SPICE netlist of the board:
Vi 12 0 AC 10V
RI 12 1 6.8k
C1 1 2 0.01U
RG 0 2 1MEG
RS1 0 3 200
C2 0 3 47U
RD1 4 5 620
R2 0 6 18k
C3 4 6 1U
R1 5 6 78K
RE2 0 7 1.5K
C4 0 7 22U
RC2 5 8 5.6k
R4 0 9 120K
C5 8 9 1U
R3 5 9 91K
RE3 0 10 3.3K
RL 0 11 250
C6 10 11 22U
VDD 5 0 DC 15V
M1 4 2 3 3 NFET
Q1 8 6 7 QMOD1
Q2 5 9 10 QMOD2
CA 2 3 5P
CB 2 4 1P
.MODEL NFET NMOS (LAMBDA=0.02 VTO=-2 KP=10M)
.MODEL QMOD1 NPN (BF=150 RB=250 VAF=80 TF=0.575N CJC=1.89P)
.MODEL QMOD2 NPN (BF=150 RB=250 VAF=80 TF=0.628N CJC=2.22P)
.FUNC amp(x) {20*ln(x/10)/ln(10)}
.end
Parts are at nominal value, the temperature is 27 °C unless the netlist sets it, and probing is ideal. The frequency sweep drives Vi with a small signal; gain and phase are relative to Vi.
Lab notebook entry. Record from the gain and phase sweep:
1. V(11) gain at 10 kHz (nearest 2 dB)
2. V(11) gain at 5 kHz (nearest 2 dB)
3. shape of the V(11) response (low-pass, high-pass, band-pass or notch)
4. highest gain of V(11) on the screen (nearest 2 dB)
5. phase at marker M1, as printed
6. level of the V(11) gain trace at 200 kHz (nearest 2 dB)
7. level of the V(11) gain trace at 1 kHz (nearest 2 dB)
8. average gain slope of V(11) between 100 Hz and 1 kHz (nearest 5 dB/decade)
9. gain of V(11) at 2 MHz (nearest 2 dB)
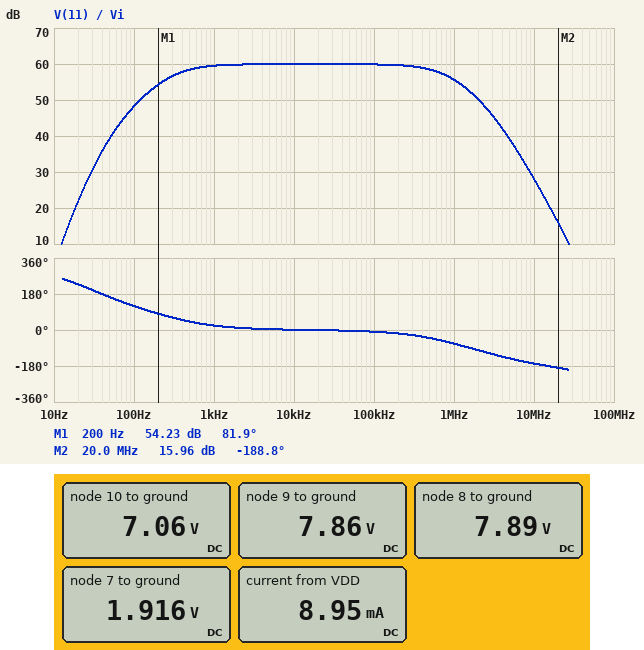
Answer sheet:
60 dB
60 dB
band-pass
60 dB
81.9 deg
60 dB
60 dB
10 dB/decade
50 dB
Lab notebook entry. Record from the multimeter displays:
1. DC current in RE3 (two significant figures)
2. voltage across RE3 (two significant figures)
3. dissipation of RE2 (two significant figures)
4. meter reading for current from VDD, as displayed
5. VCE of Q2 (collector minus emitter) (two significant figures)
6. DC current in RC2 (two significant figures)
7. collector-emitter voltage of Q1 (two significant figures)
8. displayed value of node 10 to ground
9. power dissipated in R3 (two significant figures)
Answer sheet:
2.1 mA
7.1 V
2.4 mW
8.95 mA
7.9 V
1.3 mA
6.0 V
7.06 V
560 µW
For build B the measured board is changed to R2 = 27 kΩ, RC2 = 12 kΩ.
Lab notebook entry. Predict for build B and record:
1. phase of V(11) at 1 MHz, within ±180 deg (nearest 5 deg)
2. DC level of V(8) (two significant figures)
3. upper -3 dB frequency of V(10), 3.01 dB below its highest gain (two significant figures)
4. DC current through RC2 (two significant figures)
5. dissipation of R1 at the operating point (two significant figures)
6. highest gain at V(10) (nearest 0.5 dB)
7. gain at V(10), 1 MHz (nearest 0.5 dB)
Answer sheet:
-20 deg
1.8 V
2.9 MHz
1.1 mA
2.0 mW
9.0 dB
8.5 dB
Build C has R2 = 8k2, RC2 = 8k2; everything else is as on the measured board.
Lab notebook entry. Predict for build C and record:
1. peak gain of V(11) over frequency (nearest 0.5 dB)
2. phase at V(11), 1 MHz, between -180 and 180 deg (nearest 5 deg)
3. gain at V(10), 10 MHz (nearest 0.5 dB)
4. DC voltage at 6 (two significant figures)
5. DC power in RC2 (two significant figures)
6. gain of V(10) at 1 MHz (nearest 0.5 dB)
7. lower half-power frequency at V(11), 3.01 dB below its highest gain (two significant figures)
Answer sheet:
54.5 dB
-55 deg
27.0 dB
1.4 V
1.6 mW
52.0 dB
150 Hz
